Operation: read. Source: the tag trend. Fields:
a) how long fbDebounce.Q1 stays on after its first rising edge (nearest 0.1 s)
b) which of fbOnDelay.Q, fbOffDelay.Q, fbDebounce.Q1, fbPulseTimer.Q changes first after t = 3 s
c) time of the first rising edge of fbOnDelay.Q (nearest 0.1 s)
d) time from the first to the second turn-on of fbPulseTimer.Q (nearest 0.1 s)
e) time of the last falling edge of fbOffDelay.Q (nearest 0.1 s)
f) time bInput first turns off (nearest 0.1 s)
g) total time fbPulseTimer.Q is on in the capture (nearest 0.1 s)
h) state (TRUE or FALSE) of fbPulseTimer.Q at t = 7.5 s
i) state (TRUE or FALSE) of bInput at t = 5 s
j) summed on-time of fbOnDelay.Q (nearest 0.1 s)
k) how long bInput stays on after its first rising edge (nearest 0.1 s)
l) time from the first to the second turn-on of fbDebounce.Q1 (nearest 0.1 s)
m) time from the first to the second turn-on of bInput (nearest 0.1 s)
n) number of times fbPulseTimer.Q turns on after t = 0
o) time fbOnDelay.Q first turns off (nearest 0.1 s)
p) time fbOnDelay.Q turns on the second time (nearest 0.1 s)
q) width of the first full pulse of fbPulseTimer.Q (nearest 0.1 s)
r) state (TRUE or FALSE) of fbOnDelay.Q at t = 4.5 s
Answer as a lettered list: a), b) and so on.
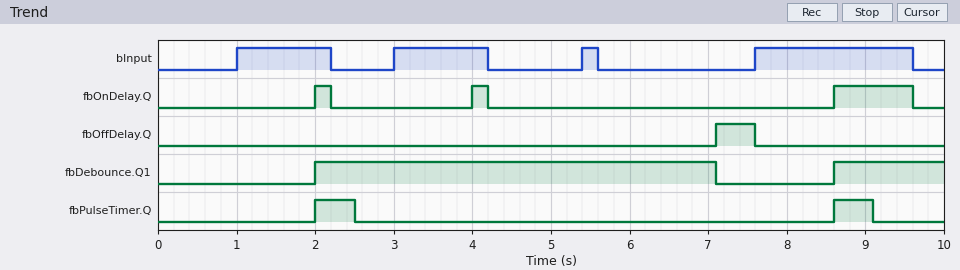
a) 5.1 s
b) fbOnDelay.Q
c) 2.0 s
d) 6.6 s
e) 7.6 s
f) 2.2 s
g) 1.0 s
h) FALSE
i) FALSE
j) 1.4 s
k) 1.2 s
l) 6.6 s
m) 2.0 s
n) 2
o) 2.2 s
p) 4.0 s
q) 0.5 s
r) FALSE
